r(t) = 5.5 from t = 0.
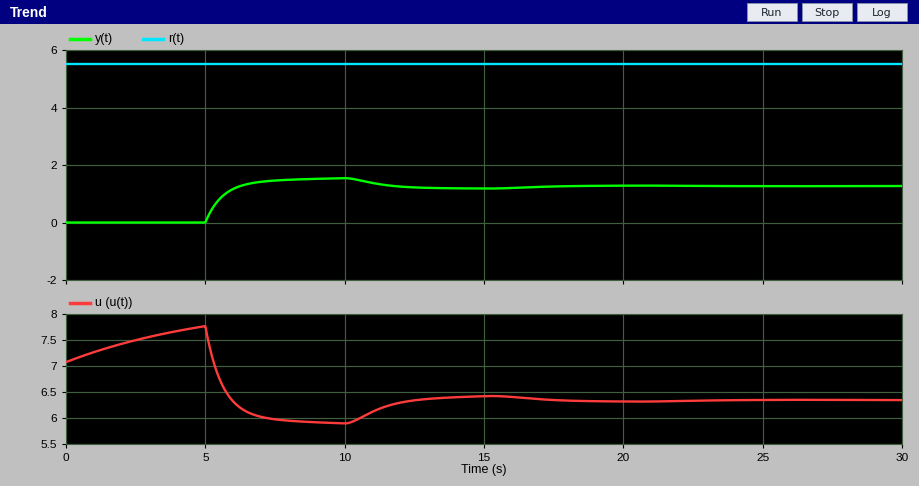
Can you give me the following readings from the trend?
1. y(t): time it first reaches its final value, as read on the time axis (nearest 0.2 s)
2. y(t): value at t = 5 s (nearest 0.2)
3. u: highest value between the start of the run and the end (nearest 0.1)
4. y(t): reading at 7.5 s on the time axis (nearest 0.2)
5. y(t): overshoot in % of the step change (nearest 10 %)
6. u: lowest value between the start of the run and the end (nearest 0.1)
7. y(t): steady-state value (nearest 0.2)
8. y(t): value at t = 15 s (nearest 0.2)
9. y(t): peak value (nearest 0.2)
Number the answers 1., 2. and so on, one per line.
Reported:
1. 6.2 s
2. 0.0
3. 7.8
4. 1.4
5. 20 %
6. 5.9
7. 1.2
8. 1.2
9. 1.6
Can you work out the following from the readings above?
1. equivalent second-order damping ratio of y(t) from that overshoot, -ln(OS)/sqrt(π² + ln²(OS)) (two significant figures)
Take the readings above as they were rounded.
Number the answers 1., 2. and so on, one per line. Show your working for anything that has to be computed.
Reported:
1. ln(0.2) = -1.609; 1.609 / sqrt(9.870 + 2.590) = 0.46
